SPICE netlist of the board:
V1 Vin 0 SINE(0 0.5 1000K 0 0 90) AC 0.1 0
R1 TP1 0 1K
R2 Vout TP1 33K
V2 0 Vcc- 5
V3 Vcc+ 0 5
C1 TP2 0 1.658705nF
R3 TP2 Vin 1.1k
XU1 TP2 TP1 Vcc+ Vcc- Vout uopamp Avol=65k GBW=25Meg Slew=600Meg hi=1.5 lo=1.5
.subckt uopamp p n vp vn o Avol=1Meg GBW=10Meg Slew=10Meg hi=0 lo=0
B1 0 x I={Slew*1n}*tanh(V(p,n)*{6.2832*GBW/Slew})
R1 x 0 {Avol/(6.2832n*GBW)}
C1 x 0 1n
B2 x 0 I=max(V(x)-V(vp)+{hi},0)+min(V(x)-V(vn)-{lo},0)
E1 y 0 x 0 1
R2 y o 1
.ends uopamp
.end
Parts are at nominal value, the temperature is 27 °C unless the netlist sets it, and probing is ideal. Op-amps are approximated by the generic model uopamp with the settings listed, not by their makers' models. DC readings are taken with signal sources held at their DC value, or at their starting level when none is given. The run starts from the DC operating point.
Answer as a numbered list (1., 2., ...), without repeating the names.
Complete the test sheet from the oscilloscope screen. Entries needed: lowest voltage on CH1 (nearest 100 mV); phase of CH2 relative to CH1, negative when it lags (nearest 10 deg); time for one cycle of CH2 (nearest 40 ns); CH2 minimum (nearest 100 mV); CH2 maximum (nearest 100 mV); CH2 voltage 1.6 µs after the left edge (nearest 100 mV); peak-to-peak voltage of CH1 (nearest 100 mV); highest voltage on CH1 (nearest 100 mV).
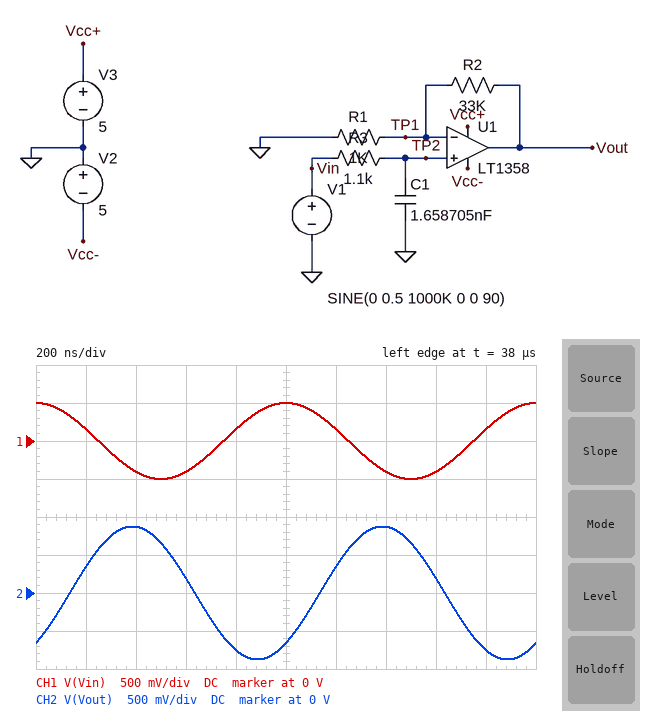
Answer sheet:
1. -500 mV
2. -140 deg
3. 1.00 µs
4. -900 mV
5. 900 mV
6. 200 mV
7. 1.0 V
8. 500 mV
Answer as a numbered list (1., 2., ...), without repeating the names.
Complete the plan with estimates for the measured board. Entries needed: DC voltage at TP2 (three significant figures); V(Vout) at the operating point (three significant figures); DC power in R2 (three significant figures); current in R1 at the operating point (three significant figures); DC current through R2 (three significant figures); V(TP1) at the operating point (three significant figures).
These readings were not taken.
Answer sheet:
1. 500 mV
2. 3.56 V
3. 362 µW
4. 105 µA
5. 105 µA
6. 105 mV
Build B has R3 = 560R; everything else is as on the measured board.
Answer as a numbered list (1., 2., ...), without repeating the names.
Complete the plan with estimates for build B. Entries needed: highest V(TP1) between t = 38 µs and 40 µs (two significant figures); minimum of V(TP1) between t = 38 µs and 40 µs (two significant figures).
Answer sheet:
1. 50 mV
2. -50 mV
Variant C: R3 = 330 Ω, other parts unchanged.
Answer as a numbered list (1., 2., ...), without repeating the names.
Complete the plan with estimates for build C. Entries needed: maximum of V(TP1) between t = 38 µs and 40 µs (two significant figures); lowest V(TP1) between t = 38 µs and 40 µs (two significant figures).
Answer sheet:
1. 83 mV
2. -83 mV
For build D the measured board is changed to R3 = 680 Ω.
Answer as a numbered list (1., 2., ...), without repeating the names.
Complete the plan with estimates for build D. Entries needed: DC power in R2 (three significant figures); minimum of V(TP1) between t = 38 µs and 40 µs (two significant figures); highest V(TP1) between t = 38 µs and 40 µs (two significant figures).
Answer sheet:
1. 362 µW
2. -41 mV
3. 41 mV
